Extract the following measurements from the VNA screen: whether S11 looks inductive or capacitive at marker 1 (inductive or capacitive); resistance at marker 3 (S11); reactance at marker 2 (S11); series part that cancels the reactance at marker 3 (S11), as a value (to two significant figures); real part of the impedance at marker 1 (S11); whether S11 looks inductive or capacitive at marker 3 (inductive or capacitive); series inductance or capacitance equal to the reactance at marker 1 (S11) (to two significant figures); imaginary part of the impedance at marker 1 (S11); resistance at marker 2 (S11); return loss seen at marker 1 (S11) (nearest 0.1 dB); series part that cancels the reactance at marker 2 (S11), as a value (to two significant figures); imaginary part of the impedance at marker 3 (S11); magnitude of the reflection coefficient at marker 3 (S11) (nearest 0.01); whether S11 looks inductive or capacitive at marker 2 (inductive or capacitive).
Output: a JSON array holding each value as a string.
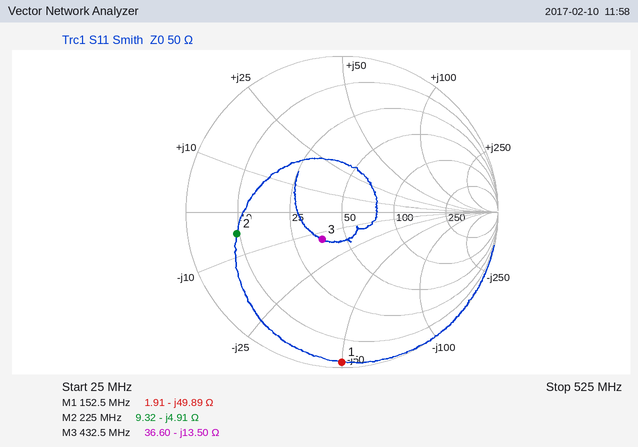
["capacitive", "36.60 Ω", "-4.91 Ω", "5.0 nH", "1.91 Ω", "capacitive", "21 pF", "-49.89 Ω", "9.32 Ω", "0.3 dB", "3.5 nH", "-13.50 Ω", "0.22", "capacitive"]
